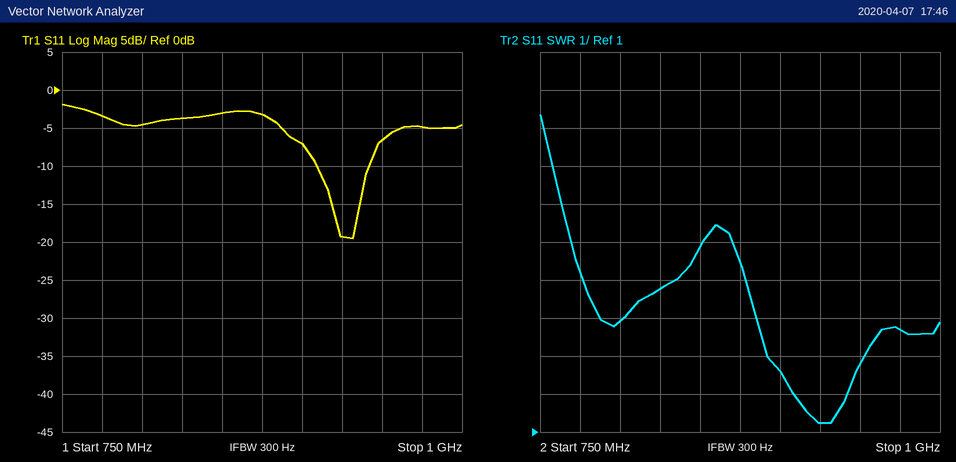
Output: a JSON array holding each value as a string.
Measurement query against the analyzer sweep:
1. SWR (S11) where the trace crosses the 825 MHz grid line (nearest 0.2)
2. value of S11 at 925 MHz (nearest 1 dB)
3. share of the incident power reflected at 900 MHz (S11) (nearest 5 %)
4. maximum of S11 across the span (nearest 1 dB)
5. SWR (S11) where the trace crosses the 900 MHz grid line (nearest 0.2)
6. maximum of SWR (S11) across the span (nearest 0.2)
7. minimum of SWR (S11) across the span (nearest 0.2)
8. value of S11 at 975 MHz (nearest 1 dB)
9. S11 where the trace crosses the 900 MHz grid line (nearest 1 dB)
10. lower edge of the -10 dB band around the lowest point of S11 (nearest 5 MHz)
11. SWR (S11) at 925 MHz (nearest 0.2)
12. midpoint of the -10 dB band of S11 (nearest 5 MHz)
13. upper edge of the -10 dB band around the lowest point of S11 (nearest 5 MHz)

["4.8", "-19 dB", "20 %", "-2 dB", "2.6", "9.4", "1.2", "-5 dB", "-7 dB", "910 MHz", "1.2", "925 MHz", "940 MHz"]
